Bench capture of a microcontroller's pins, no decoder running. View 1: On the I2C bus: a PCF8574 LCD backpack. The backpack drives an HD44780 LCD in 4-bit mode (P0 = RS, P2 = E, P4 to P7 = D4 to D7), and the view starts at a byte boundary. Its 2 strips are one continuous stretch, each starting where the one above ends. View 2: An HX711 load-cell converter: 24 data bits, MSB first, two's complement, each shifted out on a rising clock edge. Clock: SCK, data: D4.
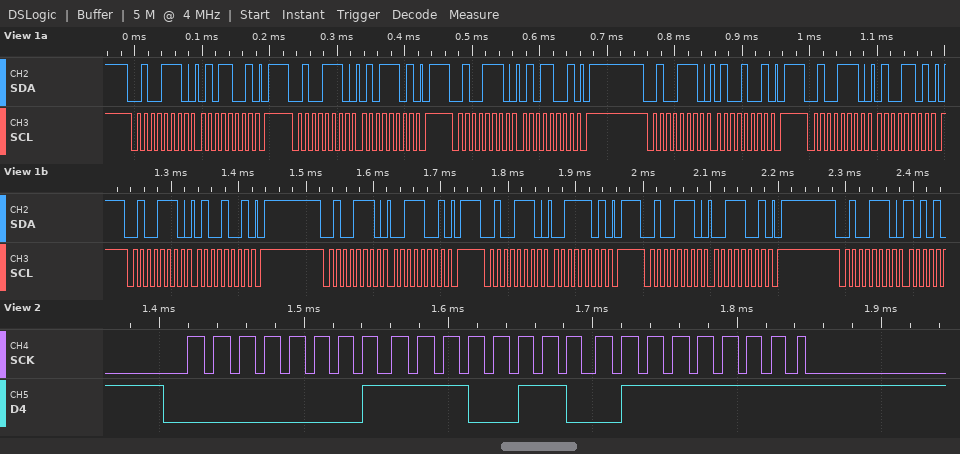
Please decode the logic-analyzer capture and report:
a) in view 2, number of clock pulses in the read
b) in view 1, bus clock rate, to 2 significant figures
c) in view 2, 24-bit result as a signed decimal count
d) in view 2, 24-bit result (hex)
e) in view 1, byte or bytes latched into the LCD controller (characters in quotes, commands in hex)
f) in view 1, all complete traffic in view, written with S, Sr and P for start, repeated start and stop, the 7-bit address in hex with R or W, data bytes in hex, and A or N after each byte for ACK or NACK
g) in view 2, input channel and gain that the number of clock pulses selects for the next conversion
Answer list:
25
100 kHz
124543
0x01E67F
'T'
S 27W A 59 A P S 27W A 5D A P S 27W A 59 A P S 27W A 49 A P S 27W A 4D A P S 27W A 49 A P S 27W A 39 A P S 27W A 3D A P S 27W A 39 A P S 27W A
channel A, gain 128
